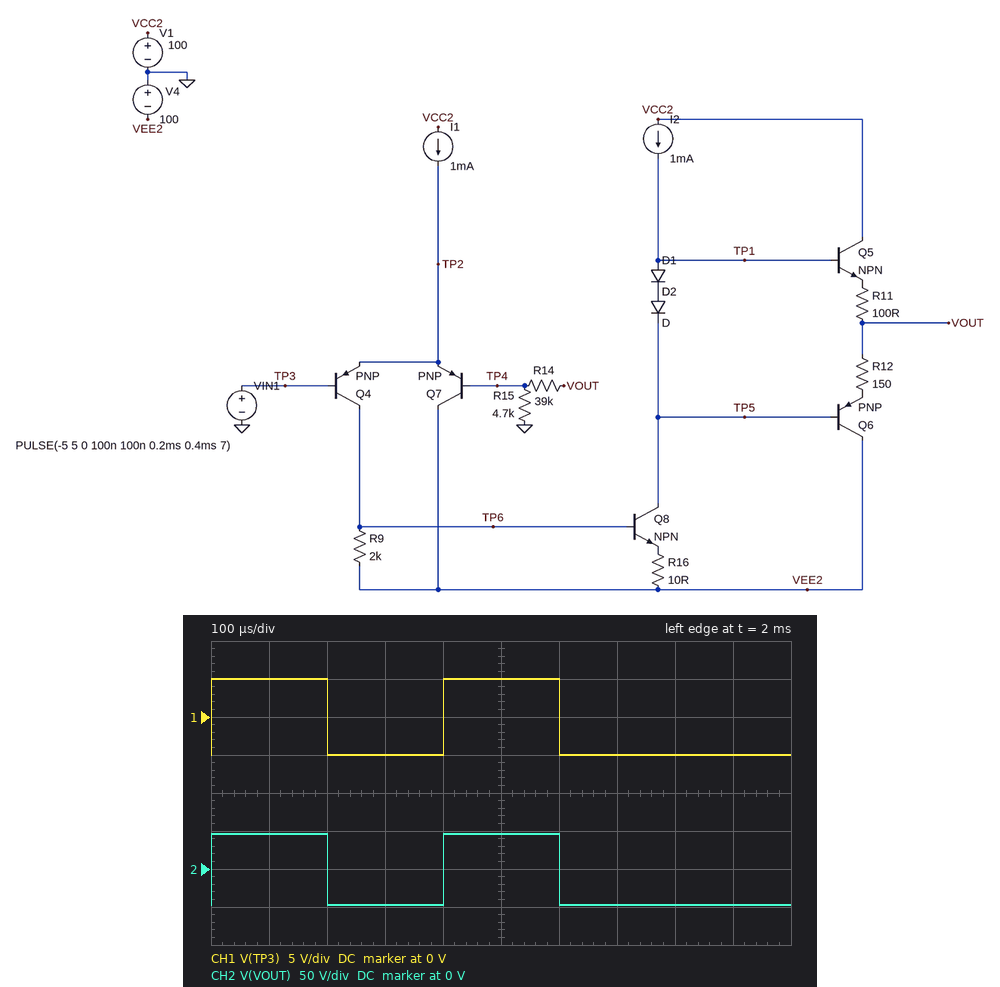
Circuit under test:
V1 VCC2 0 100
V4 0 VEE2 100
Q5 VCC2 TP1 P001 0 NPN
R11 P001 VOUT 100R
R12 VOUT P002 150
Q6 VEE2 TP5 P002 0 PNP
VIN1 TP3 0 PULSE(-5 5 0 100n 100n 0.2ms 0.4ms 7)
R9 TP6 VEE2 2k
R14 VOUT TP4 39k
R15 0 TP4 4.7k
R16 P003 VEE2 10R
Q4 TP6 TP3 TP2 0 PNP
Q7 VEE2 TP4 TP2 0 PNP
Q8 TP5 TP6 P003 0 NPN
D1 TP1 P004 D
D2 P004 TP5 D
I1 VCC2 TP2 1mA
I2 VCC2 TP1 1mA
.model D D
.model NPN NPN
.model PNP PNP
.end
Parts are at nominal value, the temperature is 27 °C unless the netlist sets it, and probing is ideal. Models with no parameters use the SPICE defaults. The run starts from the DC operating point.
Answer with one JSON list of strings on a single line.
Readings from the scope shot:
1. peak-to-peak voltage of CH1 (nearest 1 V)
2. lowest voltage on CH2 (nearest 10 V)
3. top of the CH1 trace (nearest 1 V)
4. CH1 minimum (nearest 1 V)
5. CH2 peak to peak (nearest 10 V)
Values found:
["10 V", "-50 V", "5 V", "-5 V", "90 V"]
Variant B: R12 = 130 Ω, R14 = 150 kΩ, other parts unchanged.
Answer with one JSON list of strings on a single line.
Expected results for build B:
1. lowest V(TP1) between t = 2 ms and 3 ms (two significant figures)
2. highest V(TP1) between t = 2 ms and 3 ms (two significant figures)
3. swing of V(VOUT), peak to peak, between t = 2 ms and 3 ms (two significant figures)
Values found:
["-99 V", "100 V", "200 V"]
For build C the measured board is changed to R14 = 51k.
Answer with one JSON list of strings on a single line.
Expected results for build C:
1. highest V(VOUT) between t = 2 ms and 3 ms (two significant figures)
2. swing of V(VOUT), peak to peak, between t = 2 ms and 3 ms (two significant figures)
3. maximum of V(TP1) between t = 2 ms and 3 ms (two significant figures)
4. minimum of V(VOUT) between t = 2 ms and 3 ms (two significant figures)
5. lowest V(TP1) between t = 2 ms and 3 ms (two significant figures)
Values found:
["59 V", "120 V", "60 V", "-60 V", "-59 V"]
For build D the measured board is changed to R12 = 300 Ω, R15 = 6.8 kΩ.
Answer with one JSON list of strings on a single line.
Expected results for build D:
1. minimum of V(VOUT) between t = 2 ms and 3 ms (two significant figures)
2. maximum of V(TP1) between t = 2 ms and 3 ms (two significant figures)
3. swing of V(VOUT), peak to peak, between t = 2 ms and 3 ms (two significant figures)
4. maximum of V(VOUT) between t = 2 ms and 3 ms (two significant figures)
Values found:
["-34 V", "34 V", "67 V", "33 V"]
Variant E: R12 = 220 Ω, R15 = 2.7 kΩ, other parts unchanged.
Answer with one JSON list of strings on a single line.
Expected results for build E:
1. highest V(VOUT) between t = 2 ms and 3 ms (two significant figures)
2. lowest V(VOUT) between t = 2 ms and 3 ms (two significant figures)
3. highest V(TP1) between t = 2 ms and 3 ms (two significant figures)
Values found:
["77 V", "-78 V", "78 V"]
